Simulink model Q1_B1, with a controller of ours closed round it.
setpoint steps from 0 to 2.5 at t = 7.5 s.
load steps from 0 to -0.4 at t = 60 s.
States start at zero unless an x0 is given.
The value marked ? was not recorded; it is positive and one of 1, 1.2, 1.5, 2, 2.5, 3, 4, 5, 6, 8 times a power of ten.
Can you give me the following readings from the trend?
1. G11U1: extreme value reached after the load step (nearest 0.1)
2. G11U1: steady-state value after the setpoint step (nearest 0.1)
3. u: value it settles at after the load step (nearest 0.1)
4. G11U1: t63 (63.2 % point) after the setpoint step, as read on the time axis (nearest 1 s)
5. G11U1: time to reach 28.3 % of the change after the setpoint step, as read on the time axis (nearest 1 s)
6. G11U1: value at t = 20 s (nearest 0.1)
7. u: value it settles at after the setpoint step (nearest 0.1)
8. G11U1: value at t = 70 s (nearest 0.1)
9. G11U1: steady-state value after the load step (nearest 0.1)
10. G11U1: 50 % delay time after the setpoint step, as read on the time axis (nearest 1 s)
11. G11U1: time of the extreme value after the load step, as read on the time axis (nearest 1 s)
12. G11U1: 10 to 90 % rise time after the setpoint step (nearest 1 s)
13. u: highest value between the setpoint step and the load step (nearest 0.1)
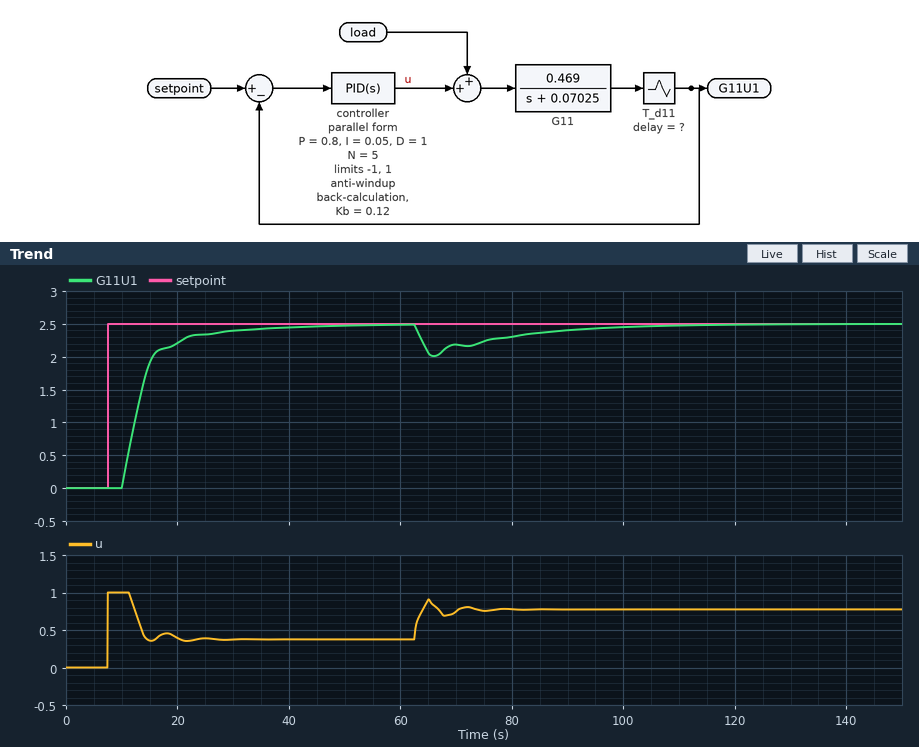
2.0
2.5
0.8
14 s
12 s
2.2
0.4
2.2
2.5
13 s
66 s
10 s
1.0
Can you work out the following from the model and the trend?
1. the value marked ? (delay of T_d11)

2.5
